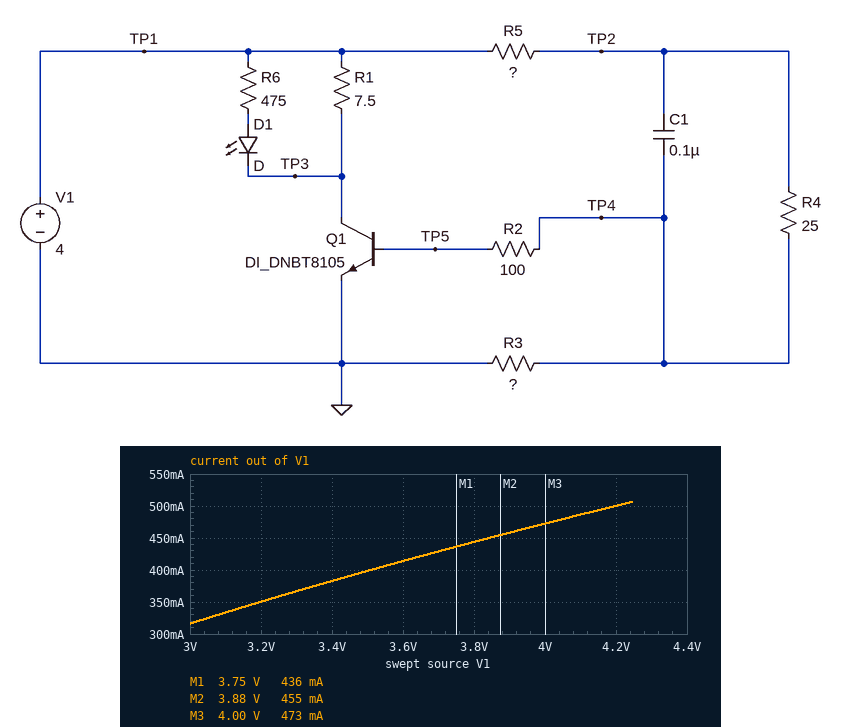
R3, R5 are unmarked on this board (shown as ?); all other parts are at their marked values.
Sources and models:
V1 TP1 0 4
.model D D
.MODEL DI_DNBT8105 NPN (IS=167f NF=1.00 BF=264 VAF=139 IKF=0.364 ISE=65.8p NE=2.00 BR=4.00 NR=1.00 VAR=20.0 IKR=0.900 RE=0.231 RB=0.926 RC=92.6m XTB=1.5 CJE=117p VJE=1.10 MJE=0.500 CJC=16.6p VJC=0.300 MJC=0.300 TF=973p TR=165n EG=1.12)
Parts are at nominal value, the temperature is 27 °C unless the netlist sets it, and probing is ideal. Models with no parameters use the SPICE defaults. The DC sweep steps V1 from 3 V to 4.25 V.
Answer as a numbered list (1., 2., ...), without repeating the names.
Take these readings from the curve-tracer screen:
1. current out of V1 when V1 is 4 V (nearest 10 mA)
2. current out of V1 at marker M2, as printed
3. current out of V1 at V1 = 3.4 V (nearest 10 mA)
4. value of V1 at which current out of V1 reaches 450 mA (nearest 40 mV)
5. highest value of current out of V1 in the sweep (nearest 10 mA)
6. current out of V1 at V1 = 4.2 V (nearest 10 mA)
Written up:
1. 470 mA
2. 455 mA
3. 380 mA
4. 3.84 V
5. 510 mA
6. 500 mA
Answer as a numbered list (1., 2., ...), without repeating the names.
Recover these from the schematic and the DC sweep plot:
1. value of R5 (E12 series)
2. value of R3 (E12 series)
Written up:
1. 180 Ω
2. 150 Ω
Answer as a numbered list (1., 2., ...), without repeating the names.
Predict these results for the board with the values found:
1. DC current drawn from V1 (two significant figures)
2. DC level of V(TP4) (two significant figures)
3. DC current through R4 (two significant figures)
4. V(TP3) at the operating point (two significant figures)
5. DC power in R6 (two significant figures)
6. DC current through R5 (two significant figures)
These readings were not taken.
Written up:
1. 470 mA
2. 1.3 V
3. 13 mA
4. 600 mV
5. 15 mW
6. 13 mA
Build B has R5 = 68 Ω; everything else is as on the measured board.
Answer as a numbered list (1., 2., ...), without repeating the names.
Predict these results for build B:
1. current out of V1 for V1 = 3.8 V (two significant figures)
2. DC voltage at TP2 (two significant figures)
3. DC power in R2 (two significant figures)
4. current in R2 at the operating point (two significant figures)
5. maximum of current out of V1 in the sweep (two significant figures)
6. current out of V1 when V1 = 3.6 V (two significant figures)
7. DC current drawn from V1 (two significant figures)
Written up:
1. 500 mA
2. 2.5 V
3. 10 mW
4. 10 mA
5. 560 mA
6. 470 mA
7. 530 mA
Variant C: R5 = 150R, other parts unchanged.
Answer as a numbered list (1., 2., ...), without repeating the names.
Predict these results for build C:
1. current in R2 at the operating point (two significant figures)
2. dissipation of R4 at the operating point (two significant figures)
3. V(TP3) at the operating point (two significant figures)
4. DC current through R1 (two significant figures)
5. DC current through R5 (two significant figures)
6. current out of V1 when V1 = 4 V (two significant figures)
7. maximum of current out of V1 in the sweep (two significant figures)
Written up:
1. 5.3 mA
2. 5.4 mW
3. 340 mV
4. 490 mA
5. 15 mA
6. 510 mA
7. 540 mA
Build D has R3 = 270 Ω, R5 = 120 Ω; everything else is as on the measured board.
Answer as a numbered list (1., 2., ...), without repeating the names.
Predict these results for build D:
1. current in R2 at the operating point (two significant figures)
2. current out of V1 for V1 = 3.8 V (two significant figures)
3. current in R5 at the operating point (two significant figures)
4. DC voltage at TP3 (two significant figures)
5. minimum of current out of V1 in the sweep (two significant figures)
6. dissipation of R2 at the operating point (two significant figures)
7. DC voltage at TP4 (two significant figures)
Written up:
1. 8.8 mA
2. 490 mA
3. 15 mA
4. 280 mV
5. 380 mA
6. 7.7 mW
7. 1.8 V
